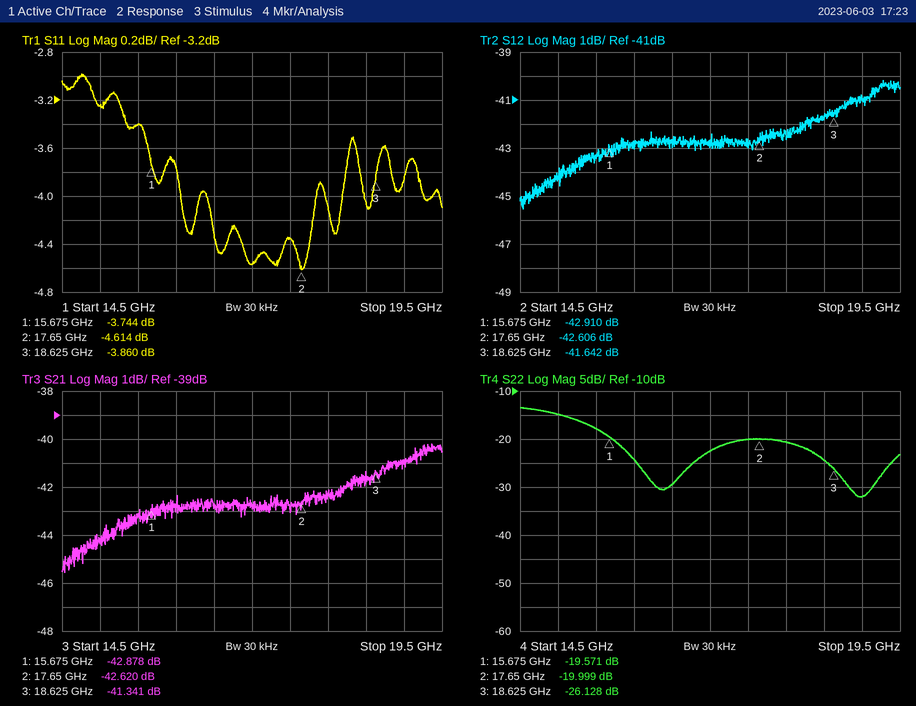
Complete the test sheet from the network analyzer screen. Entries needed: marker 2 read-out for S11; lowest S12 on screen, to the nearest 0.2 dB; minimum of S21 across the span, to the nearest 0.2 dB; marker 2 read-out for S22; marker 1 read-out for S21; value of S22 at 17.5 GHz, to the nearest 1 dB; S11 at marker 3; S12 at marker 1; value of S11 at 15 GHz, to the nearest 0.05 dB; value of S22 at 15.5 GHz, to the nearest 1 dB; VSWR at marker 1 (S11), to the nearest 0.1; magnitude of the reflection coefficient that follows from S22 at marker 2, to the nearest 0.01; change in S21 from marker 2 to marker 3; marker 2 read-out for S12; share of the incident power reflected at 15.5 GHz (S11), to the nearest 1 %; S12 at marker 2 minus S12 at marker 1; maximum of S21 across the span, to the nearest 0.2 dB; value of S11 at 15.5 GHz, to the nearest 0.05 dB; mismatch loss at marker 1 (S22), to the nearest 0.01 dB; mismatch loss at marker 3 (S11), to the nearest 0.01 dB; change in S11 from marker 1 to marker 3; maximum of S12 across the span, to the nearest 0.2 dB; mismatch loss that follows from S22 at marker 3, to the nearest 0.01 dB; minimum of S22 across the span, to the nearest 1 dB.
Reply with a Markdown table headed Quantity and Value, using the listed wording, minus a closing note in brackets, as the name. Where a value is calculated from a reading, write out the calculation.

| Quantity | Value |
|---|---|
| marker 2 read-out for S11 | -4.614 dB |
| lowest S12 on screen, to the nearest 0.2 dB | -45.6 dB |
| minimum of S21 across the span, to the nearest 0.2 dB | -45.6 dB |
| marker 2 read-out for S22 | -19.999 dB |
| marker 1 read-out for S21 | -42.878 dB |
| value of S22 at 17.5 GHz, to the nearest 1 dB | -20 dB |
| S11 at marker 3 | -3.860 dB |
| S12 at marker 1 | -42.910 dB |
| value of S11 at 15 GHz, to the nearest 0.05 dB | -3.25 dB |
| value of S22 at 15.5 GHz, to the nearest 1 dB | -18 dB |
| VSWR at marker 1 (S11), to the nearest 0.1 | (1 + 0.6498)/(1 − 0.6498) ≈ 4.7 |
| magnitude of the reflection coefficient that follows from S22 at marker 2, to the nearest 0.01 | 10^(-19.999/20) ≈ 0.10 |
| change in S21 from marker 2 to marker 3 | -41.341 − (-42.62) = 1.279 dB |
| marker 2 read-out for S12 | -42.606 dB |
| share of the incident power reflected at 15.5 GHz (S11), to the nearest 1 % | 10^(-3.4/10) ≈ 46 % |
| S12 at marker 2 minus S12 at marker 1 | -42.606 − (-42.91) = 0.304 dB |
| maximum of S21 across the span, to the nearest 0.2 dB | -40.2 dB |
| value of S11 at 15.5 GHz, to the nearest 0.05 dB | -3.40 dB |
| mismatch loss at marker 1 (S22), to the nearest 0.01 dB | −10 log10(1 − 10^(-19.571/10)) ≈ 0.05 dB |
| mismatch loss at marker 3 (S11), to the nearest 0.01 dB | −10 log10(1 − 10^(-3.86/10)) ≈ 2.30 dB |
| change in S11 from marker 1 to marker 3 | -3.86 − (-3.744) = -0.116 dB |
| maximum of S12 across the span, to the nearest 0.2 dB | -40.2 dB |
| mismatch loss that follows from S22 at marker 3, to the nearest 0.01 dB | −10 log10(1 − 10^(-26.128/10)) ≈ 0.01 dB |
| minimum of S22 across the span, to the nearest 1 dB | -32 dB |
